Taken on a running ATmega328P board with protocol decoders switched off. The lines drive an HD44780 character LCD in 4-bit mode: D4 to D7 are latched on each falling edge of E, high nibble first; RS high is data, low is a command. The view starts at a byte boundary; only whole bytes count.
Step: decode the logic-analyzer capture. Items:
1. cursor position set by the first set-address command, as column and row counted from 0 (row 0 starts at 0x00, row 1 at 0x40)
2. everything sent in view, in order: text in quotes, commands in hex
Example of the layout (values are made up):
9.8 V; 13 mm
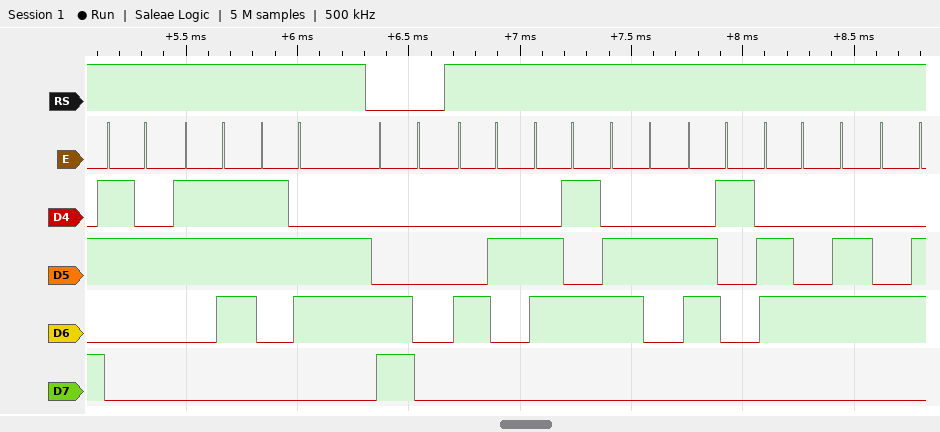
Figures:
column 0, row 1; "276" 0xC0 "Bebadd"
